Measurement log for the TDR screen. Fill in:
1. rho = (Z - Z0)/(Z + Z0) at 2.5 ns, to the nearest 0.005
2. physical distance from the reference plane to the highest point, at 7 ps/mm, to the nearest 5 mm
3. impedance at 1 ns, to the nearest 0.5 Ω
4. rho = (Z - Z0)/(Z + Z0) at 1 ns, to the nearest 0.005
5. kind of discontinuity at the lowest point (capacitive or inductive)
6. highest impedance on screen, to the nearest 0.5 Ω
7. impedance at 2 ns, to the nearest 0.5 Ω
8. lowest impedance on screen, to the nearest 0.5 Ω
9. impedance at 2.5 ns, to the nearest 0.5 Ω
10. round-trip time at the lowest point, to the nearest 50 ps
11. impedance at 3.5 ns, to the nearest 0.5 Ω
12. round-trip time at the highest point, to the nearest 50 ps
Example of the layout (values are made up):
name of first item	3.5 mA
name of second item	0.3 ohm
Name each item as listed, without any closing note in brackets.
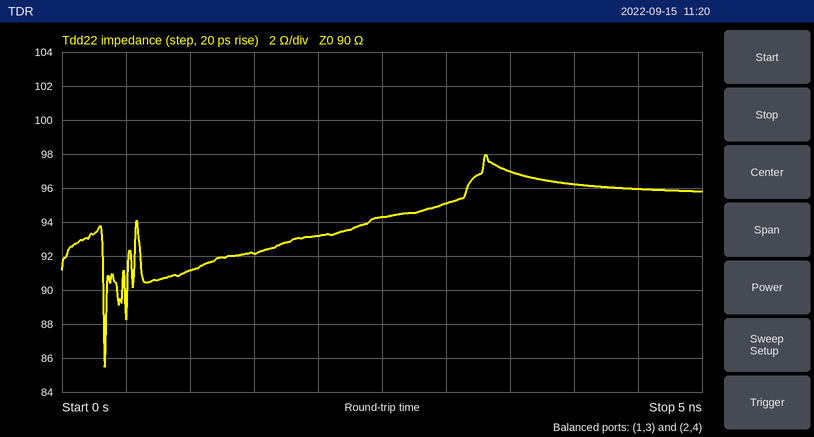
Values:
rho = (Z - Z0)/(Z + Z0) at 2.5 ns, to the nearest 0.005	+0.025
physical distance from the reference plane to the highest point, at 7 ps/mm, to the nearest 5 mm	235 mm
impedance at 1 ns, to the nearest 0.5 Ω	91.0 Ω
rho = (Z - Z0)/(Z + Z0) at 1 ns, to the nearest 0.005	+0.005
kind of discontinuity at the lowest point	capacitive
highest impedance on screen, to the nearest 0.5 Ω	98.0 Ω
impedance at 2 ns, to the nearest 0.5 Ω	93.0 Ω
lowest impedance on screen, to the nearest 0.5 Ω	85.5 Ω
impedance at 2.5 ns, to the nearest 0.5 Ω	94.5 Ω
round-trip time at the lowest point, to the nearest 50 ps	350 ps
impedance at 3.5 ns, to the nearest 0.5 Ω	97.0 Ω
round-trip time at the highest point, to the nearest 50 ps	3.30 ns
